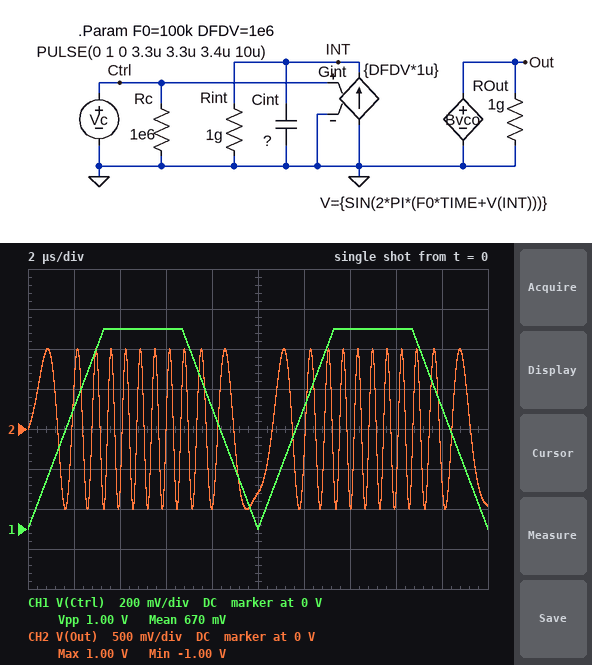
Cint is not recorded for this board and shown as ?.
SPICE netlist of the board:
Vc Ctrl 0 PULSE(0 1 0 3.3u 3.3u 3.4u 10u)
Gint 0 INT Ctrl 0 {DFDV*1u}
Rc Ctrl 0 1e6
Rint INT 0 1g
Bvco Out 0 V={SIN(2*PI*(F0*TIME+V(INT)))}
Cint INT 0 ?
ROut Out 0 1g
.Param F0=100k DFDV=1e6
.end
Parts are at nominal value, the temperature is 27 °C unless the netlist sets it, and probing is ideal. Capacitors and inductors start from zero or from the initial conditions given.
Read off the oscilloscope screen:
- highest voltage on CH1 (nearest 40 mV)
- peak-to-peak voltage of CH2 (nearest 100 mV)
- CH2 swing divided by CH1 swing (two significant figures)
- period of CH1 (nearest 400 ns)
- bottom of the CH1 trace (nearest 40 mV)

1.00 V
2.0 V
2.0
10.0 µs
0 V
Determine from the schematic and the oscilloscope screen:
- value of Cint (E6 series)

680 nF
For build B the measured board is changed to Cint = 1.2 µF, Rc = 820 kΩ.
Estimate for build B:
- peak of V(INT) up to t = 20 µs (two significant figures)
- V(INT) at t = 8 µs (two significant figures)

11 V
5.1 V
